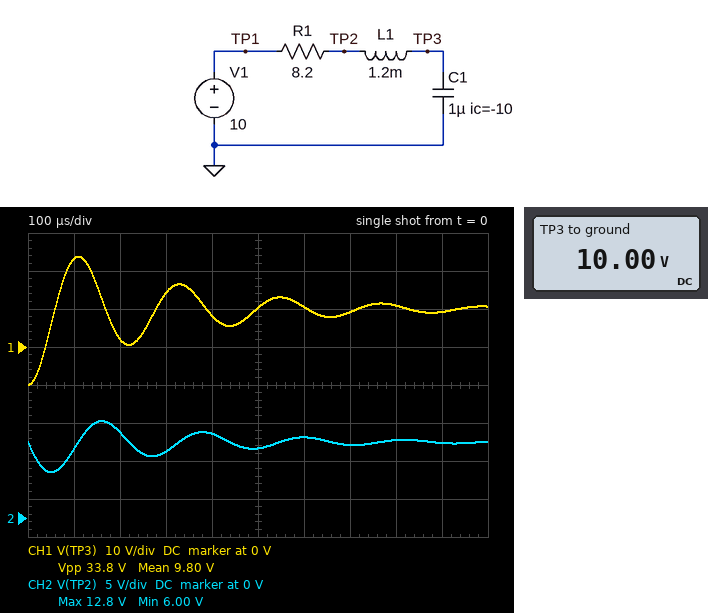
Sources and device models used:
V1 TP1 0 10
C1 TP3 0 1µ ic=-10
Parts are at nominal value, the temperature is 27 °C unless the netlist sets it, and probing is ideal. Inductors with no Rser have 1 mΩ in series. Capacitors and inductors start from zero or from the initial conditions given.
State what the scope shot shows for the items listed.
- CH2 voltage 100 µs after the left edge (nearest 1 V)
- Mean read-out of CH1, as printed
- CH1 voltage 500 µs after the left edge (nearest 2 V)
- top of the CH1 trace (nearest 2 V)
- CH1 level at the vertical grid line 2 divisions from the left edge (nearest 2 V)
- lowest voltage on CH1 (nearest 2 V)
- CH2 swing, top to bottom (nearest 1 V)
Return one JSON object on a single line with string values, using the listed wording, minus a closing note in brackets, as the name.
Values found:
{"CH2 voltage 100 µs after the left edge": "9 V", "Mean read-out of CH1, as printed": "9.80 V", "CH1 voltage 500 µs after the left edge": "10 V", "top of the CH1 trace": "24 V", "CH1 level at the vertical grid line 2 divisions from the left edge": "2 V", "lowest voltage on CH1": "-10 V", "CH2 swing, top to bottom": "7 V"}
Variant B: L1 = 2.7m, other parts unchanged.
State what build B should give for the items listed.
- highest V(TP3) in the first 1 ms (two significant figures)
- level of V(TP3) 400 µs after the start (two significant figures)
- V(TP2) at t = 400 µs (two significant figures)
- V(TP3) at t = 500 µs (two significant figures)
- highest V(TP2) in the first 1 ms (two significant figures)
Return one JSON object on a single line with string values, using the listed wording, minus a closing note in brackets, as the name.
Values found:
{"highest V(TP3) in the first 1 ms": "26 V", "level of V(TP3) 400 µs after the start": "7.2 V", "V(TP2) at t = 400 µs": "8.3 V", "V(TP3) at t = 500 µs": "19 V", "highest V(TP2) in the first 1 ms": "12 V"}
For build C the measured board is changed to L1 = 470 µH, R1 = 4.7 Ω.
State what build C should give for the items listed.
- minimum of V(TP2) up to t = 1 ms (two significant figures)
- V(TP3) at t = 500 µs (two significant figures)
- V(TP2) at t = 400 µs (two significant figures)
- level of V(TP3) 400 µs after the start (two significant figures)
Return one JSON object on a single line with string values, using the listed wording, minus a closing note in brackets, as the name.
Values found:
{"minimum of V(TP2) up to t = 1 ms": "6.3 V", "V(TP3) at t = 500 µs": "11 V", "V(TP2) at t = 400 µs": "10 V", "level of V(TP3) 400 µs after the start": "7.8 V"}
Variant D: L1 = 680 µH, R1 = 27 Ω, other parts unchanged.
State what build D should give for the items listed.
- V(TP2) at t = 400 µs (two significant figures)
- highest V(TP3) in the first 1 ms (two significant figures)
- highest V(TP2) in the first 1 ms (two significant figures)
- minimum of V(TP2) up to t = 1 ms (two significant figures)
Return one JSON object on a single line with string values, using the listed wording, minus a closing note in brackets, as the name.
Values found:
{"V(TP2) at t = 400 µs": "10 V", "highest V(TP3) in the first 1 ms": "13 V", "highest V(TP2) in the first 1 ms": "12 V", "minimum of V(TP2) up to t = 1 ms": "-1.1 V"}
